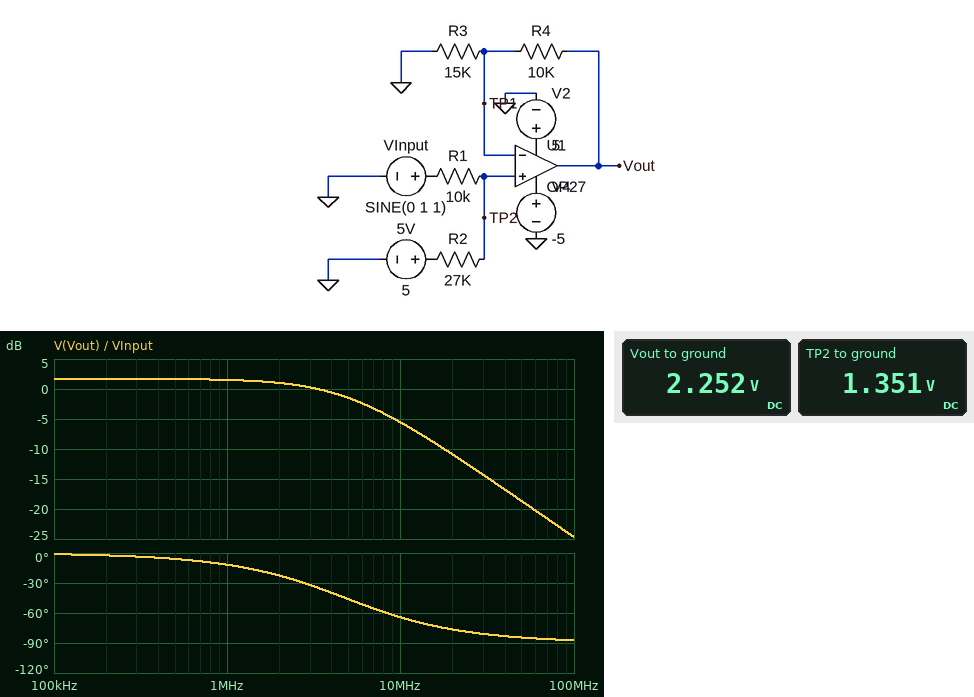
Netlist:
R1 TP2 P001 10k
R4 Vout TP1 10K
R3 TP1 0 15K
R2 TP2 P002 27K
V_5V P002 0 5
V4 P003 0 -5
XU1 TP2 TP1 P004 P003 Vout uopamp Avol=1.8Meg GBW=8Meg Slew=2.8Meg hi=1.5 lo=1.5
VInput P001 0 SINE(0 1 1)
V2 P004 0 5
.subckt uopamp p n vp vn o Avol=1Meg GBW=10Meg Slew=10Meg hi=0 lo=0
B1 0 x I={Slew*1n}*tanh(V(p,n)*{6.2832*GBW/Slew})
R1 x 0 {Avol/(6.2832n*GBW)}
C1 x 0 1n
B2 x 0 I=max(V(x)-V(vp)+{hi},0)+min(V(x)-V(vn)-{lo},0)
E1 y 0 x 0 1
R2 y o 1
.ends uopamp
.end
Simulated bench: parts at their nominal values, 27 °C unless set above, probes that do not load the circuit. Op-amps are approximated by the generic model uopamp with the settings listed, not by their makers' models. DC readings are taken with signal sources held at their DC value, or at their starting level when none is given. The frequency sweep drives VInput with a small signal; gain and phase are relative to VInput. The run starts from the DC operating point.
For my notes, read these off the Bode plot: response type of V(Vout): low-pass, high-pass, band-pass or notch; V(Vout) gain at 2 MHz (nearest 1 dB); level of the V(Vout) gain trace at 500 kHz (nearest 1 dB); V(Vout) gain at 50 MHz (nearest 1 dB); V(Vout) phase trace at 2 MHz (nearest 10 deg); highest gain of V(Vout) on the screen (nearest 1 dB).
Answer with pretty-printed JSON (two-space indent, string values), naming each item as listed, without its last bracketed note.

{
  "response type of V(Vout): low-pass, high-pass, band-pass or notch": "low-pass",
  "V(Vout) gain at 2 MHz": "1 dB",
  "level of the V(Vout) gain trace at 500 kHz": "2 dB",
  "V(Vout) gain at 50 MHz": "-19 dB",
  "V(Vout) phase trace at 2 MHz": "-20 deg",
  "highest gain of V(Vout) on the screen": "2 dB"
}
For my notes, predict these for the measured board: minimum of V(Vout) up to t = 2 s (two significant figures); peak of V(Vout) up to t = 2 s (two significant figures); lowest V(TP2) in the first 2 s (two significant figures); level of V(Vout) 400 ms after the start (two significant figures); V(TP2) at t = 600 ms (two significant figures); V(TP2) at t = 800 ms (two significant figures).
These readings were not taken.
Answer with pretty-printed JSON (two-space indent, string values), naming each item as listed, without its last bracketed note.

{
  "minimum of V(Vout) up to t = 2 s": "1.0 V",
  "peak of V(Vout) up to t = 2 s": "3.5 V",
  "lowest V(TP2) in the first 2 s": "620 mV",
  "level of V(Vout) 400 ms after the start": "3.0 V",
  "V(TP2) at t = 600 ms": "920 mV",
  "V(TP2) at t = 800 ms": "660 mV"
}
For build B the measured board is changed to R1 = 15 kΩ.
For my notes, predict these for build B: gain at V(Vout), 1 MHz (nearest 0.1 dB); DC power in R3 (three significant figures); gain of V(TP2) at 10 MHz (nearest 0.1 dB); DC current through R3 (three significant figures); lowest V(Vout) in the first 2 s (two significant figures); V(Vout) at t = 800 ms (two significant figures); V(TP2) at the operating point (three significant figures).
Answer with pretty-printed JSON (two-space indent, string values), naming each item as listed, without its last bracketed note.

{
  "gain at V(Vout), 1 MHz": "0.4 dB",
  "DC power in R3": "213 µW",
  "gain of V(TP2) at 10 MHz": "-3.8 dB",
  "DC current through R3": "119 µA",
  "lowest V(Vout) in the first 2 s": "1.9 V",
  "V(Vout) at t = 800 ms": "2.0 V",
  "V(TP2) at the operating point": "1.79 V"
}
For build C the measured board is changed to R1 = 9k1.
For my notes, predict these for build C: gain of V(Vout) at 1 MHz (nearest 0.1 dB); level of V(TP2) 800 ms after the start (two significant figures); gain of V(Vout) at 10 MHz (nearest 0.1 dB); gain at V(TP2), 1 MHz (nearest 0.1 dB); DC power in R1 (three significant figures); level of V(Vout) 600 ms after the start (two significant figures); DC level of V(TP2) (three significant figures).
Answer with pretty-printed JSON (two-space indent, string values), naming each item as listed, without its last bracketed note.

{
  "gain of V(Vout) at 1 MHz": "1.7 dB",
  "level of V(TP2) 800 ms after the start": "550 mV",
  "gain of V(Vout) at 10 MHz": "-5.4 dB",
  "gain at V(TP2), 1 MHz": "-2.5 dB",
  "DC power in R1": "175 µW",
  "level of V(Vout) 600 ms after the start": "1.4 V",
  "DC level of V(TP2)": "1.26 V"
}
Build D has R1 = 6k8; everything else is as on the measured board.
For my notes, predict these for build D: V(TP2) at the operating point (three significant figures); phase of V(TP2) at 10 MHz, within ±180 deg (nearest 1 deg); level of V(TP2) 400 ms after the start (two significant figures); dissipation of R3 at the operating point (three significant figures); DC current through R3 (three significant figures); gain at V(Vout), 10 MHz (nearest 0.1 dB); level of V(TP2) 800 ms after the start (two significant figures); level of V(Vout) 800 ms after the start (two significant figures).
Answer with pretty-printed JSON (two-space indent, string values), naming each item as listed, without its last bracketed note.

{
  "V(TP2) at the operating point": "1.01 V",
  "phase of V(TP2) at 10 MHz, within ±180 deg": "0 deg",
  "level of V(TP2) 400 ms after the start": "1.5 V",
  "dissipation of R3 at the operating point": "67.5 µW",
  "DC current through R3": "67.1 µA",
  "gain at V(Vout), 10 MHz": "-4.8 dB",
  "level of V(TP2) 800 ms after the start": "250 mV",
  "level of V(Vout) 800 ms after the start": "410 mV"
}
